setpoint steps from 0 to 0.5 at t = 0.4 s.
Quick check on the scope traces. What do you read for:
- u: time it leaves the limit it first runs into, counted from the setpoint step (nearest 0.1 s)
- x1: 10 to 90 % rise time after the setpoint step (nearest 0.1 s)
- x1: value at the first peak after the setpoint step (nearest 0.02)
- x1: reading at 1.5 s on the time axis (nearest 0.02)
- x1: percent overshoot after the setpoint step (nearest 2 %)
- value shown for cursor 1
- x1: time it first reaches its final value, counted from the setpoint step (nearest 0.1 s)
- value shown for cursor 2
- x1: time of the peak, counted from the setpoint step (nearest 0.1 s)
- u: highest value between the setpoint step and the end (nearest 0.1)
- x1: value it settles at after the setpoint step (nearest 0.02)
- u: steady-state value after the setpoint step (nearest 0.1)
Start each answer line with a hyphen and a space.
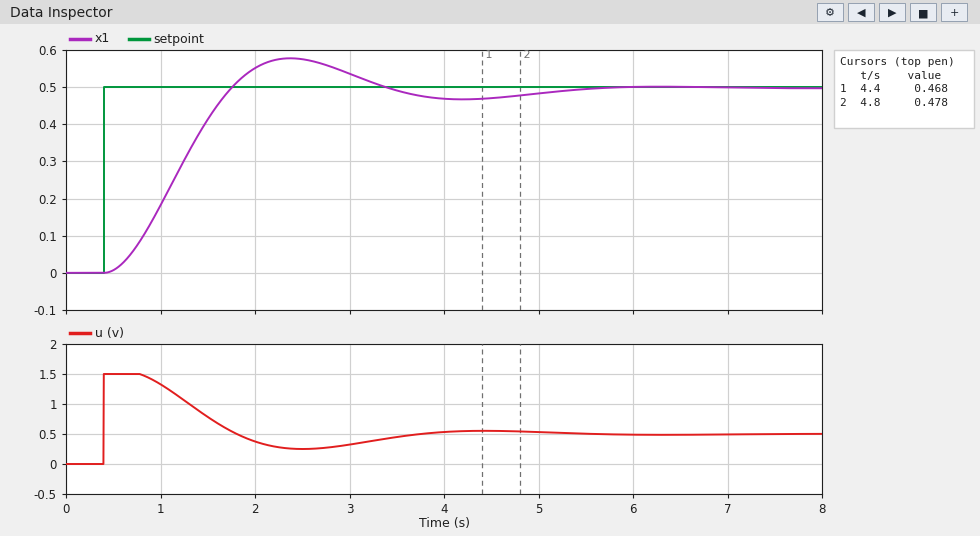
- 0.4 s
- 0.9 s
- 0.58
- 0.42
- 16 %
- 0.468
- 1.4 s
- 0.478
- 2.0 s
- 1.5
- 0.50
- 0.5
